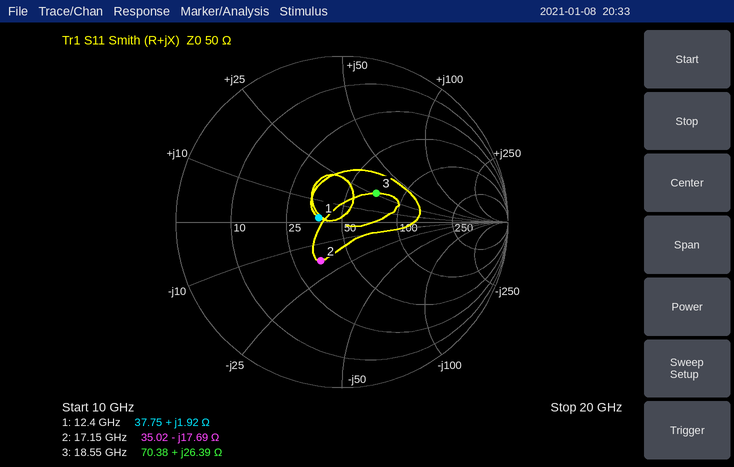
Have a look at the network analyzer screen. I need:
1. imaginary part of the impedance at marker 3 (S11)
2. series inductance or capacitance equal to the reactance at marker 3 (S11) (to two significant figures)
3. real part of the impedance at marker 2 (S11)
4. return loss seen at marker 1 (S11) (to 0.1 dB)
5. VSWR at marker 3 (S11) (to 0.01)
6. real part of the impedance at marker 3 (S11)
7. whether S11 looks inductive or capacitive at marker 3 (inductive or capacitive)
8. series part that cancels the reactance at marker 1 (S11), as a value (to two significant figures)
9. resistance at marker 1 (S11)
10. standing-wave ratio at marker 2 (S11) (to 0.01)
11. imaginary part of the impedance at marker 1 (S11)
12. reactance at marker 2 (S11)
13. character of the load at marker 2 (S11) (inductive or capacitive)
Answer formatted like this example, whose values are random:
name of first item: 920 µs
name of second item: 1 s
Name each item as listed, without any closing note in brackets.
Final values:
imaginary part of the impedance at marker 3: +26.39 Ω
series inductance or capacitance equal to the reactance at marker 3 (S11): 230 pH
real part of the impedance at marker 2: 35.02 Ω
return loss seen at marker 1 (S11): 17.0 dB
VSWR at marker 3 (S11): 1.74
real part of the impedance at marker 3: 70.38 Ω
whether S11 looks inductive or capacitive at marker 3: inductive
series part that cancels the reactance at marker 1 (S11), as a value: 6.7 pF
resistance at marker 1: 37.75 Ω
standing-wave ratio at marker 2 (S11): 1.73
imaginary part of the impedance at marker 1: +1.92 Ω
reactance at marker 2: -17.69 Ω
character of the load at marker 2 (S11): capacitive
